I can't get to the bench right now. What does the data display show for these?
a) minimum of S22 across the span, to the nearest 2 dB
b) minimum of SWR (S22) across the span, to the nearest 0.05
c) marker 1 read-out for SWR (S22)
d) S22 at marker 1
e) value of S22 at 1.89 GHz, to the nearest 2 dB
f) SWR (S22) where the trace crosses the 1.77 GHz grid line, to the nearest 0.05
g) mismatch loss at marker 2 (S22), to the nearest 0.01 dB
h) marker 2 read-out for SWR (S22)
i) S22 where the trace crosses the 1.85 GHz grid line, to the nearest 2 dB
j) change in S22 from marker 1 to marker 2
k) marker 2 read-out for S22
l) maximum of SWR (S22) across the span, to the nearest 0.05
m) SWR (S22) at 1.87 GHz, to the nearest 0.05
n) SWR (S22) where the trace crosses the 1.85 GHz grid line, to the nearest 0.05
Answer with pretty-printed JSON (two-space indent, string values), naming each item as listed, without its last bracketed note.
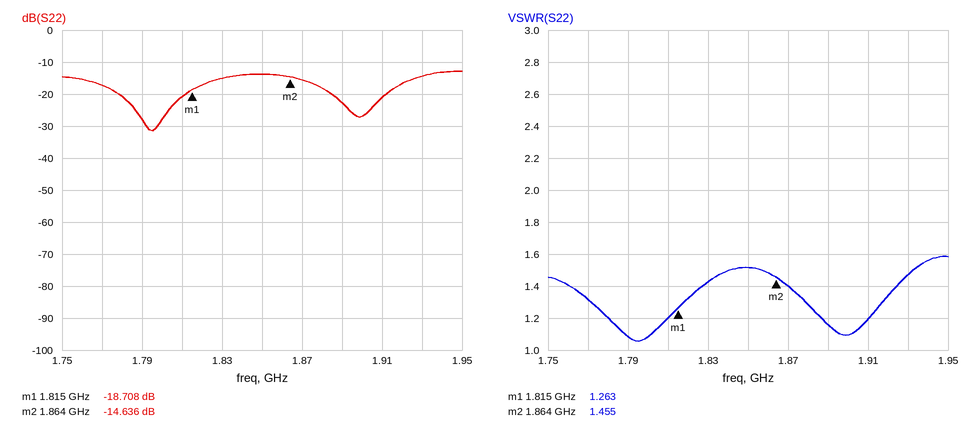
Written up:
{
  "minimum of S22 across the span, to the nearest 2 dB": "-32 dB",
  "minimum of SWR (S22) across the span, to the nearest 0.05": "1.05",
  "marker 1 read-out for SWR": "1.263",
  "S22 at marker 1": "-18.708 dB",
  "value of S22 at 1.89 GHz, to the nearest 2 dB": "-22 dB",
  "SWR (S22) where the trace crosses the 1.77 GHz grid line, to the nearest 0.05": "1.30",
  "mismatch loss at marker 2 (S22), to the nearest 0.01 dB": "0.15 dB",
  "marker 2 read-out for SWR": "1.455",
  "S22 where the trace crosses the 1.85 GHz grid line, to the nearest 2 dB": "-14 dB",
  "change in S22 from marker 1 to marker 2": "4.072 dB",
  "marker 2 read-out for S22": "-14.636 dB",
  "maximum of SWR (S22) across the span, to the nearest 0.05": "1.60",
  "SWR (S22) at 1.87 GHz, to the nearest 0.05": "1.40",
  "SWR (S22) where the trace crosses the 1.85 GHz grid line, to the nearest 0.05": "1.50"
}
